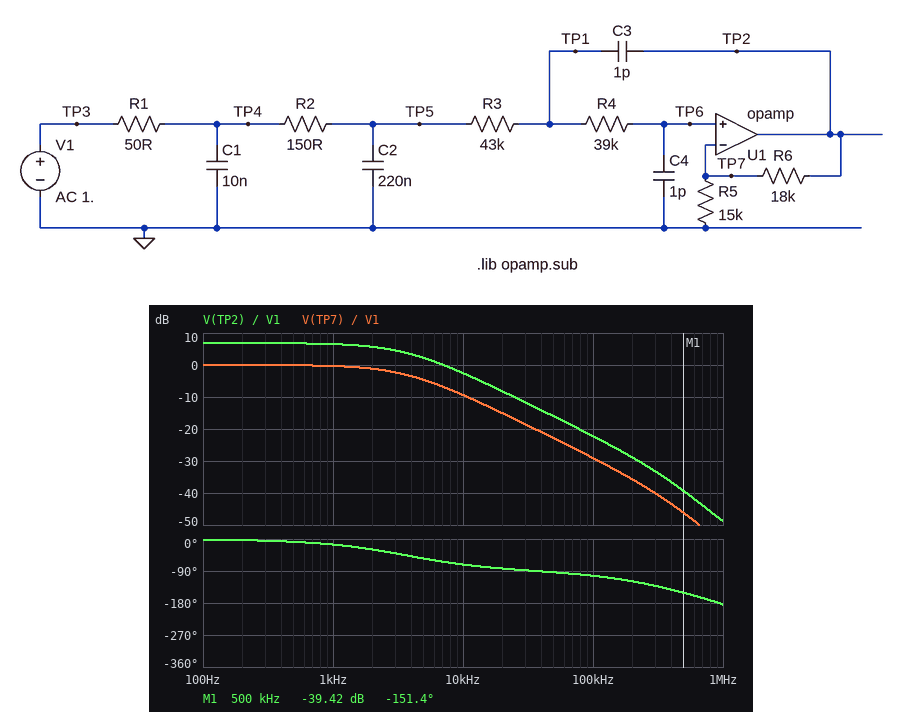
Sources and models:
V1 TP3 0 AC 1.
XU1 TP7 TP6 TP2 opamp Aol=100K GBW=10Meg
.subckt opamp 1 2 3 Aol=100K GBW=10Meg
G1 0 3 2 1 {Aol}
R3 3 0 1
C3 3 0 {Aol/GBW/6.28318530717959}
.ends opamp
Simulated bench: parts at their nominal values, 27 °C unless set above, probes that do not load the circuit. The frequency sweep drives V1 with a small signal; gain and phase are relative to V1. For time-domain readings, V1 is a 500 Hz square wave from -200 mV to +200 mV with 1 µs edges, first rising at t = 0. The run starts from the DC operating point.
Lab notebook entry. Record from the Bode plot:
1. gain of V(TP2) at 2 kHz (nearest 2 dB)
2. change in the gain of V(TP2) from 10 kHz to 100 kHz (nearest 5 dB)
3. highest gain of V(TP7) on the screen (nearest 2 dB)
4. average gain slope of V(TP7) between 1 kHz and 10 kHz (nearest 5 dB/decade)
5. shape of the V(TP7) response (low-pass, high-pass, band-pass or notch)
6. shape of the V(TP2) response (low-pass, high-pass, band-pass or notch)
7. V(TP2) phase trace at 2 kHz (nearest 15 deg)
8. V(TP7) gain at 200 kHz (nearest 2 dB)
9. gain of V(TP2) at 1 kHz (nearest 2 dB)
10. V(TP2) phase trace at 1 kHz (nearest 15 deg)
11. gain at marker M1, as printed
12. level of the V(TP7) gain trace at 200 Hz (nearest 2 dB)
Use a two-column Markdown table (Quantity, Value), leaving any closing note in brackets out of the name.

| Quantity | Value |
|---|---|
| gain of V(TP2) at 2 kHz | 6 dB |
| change in the gain of V(TP2) from 10 kHz to 100 kHz | -20 dB |
| highest gain of V(TP7) on the screen | 0 dB |
| average gain slope of V(TP7) between 1 kHz and 10 kHz | -10 dB/decade |
| shape of the V(TP7) response | low-pass |
| shape of the V(TP2) response | low-pass |
| V(TP2) phase trace at 2 kHz | -30 deg |
| V(TP7) gain at 200 kHz | -36 dB |
| gain of V(TP2) at 1 kHz | 6 dB |
| V(TP2) phase trace at 1 kHz | -15 deg |
| gain at marker M1, as printed | -39.42 dB |
| level of the V(TP7) gain trace at 200 Hz | 0 dB |
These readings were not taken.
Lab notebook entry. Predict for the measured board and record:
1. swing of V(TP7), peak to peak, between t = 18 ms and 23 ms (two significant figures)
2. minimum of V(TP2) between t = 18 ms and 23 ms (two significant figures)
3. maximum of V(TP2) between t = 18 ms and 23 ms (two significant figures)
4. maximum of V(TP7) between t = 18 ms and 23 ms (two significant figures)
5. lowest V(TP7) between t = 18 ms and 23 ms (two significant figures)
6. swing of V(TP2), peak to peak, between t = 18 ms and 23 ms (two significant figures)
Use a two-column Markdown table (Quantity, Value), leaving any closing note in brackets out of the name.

| Quantity | Value |
|---|---|
| swing of V(TP7), peak to peak, between t = 18 ms and 23 ms | 400 mV |
| minimum of V(TP2) between t = 18 ms and 23 ms | -440 mV |
| maximum of V(TP2) between t = 18 ms and 23 ms | 440 mV |
| maximum of V(TP7) between t = 18 ms and 23 ms | 200 mV |
| lowest V(TP7) between t = 18 ms and 23 ms | -200 mV |
| swing of V(TP2), peak to peak, between t = 18 ms and 23 ms | 880 mV |
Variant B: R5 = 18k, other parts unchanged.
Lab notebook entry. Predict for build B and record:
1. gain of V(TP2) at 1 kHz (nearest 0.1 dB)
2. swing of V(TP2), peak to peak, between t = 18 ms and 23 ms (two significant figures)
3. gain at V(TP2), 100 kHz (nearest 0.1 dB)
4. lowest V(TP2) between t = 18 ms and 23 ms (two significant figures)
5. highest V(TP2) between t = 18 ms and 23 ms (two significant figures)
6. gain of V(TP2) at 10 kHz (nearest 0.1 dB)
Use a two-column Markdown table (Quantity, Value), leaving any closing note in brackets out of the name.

| Quantity | Value |
|---|---|
| gain of V(TP2) at 1 kHz | 5.7 dB |
| swing of V(TP2), peak to peak, between t = 18 ms and 23 ms | 800 mV |
| gain at V(TP2), 100 kHz | -23.1 dB |
| lowest V(TP2) between t = 18 ms and 23 ms | -400 mV |
| highest V(TP2) between t = 18 ms and 23 ms | 400 mV |
| gain of V(TP2) at 10 kHz | -3.4 dB |
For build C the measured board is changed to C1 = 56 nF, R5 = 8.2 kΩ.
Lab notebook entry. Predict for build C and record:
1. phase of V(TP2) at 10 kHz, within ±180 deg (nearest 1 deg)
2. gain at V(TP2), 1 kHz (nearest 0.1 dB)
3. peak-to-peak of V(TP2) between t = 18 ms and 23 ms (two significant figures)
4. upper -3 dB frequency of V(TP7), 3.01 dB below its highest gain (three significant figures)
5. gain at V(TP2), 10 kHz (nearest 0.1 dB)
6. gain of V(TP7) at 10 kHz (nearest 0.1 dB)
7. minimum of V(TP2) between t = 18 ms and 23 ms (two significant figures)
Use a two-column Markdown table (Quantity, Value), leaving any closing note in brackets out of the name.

| Quantity | Value |
|---|---|
| phase of V(TP2) at 10 kHz, within ±180 deg | -78 deg |
| gain at V(TP2), 1 kHz | 9.8 dB |
| peak-to-peak of V(TP2) between t = 18 ms and 23 ms | 1.3 V |
| upper -3 dB frequency of V(TP7), 3.01 dB below its highest gain | 3.55 kHz |
| gain at V(TP2), 10 kHz | 0.5 dB |
| gain of V(TP7) at 10 kHz | -9.6 dB |
| minimum of V(TP2) between t = 18 ms and 23 ms | -640 mV |
